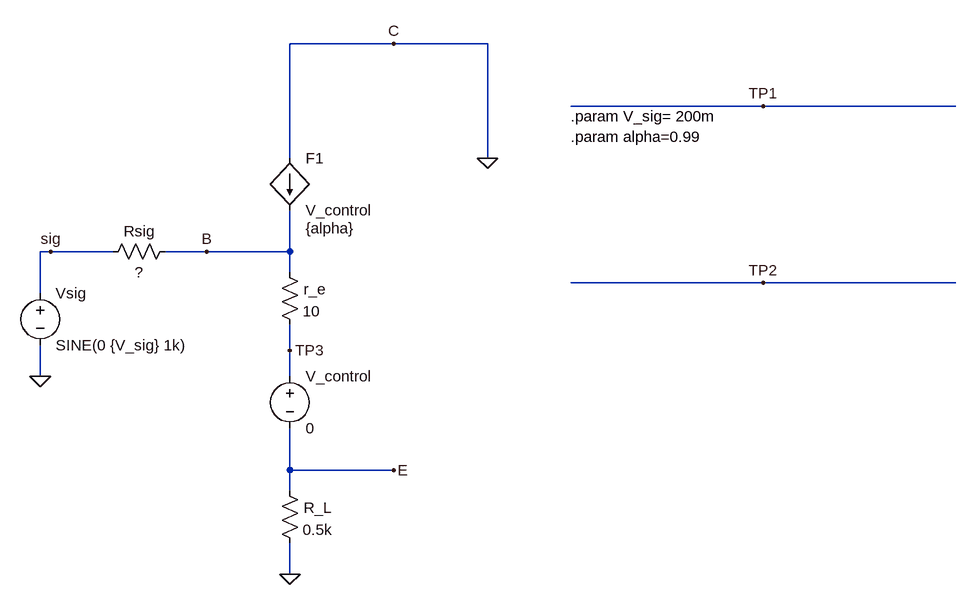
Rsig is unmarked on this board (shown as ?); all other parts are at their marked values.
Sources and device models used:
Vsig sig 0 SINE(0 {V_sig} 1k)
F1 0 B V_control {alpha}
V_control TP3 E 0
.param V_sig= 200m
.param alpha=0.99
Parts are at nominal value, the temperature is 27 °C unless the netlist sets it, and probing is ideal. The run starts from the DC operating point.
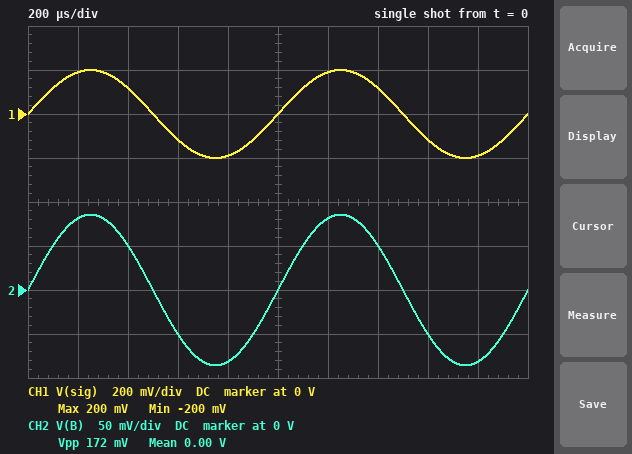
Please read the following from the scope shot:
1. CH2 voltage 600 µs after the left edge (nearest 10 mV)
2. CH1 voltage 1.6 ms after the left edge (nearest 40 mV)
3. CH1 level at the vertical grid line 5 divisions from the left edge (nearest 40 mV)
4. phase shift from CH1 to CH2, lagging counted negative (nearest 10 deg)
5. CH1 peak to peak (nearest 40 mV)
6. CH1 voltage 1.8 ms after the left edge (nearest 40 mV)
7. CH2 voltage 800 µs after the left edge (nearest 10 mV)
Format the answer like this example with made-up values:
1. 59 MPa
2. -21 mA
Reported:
1. -50 mV
2. -120 mV
3. 0 V
4. 0 deg
5. 400 mV
6. -200 mV
7. -80 mV
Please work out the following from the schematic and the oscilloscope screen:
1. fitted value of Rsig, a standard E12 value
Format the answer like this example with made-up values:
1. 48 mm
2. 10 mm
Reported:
1. 68 kΩ
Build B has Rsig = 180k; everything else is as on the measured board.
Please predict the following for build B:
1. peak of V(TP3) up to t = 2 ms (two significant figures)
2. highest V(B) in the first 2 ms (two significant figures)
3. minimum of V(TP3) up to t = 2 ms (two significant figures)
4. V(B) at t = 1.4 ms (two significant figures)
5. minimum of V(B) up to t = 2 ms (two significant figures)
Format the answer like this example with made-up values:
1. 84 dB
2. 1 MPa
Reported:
1. 43 mV
2. 44 mV
3. -43 mV
4. 26 mV
5. -44 mV
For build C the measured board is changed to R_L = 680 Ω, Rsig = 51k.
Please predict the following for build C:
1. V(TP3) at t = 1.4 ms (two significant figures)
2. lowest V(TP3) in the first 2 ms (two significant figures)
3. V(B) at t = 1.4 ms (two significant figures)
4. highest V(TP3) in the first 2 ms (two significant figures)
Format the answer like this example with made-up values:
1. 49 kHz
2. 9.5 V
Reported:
1. 67 mV
2. -110 mV
3. 68 mV
4. 110 mV
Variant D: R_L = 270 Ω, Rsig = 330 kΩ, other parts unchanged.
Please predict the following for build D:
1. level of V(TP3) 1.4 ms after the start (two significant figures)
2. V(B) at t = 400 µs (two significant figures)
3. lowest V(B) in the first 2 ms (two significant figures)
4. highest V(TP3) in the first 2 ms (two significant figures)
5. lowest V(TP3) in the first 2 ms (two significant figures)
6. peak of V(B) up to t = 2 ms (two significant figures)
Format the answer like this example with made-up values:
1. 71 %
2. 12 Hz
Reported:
1. 8.9 mV
2. 9.2 mV
3. -16 mV
4. 15 mV
5. -15 mV
6. 16 mV
